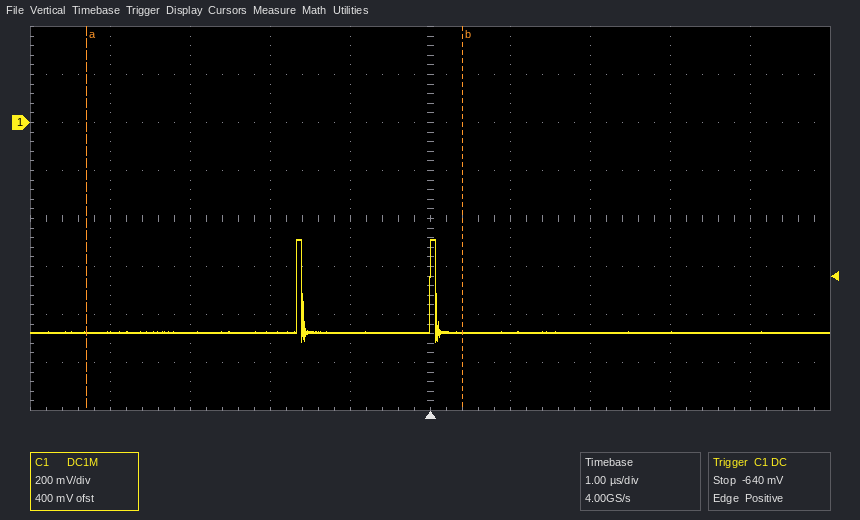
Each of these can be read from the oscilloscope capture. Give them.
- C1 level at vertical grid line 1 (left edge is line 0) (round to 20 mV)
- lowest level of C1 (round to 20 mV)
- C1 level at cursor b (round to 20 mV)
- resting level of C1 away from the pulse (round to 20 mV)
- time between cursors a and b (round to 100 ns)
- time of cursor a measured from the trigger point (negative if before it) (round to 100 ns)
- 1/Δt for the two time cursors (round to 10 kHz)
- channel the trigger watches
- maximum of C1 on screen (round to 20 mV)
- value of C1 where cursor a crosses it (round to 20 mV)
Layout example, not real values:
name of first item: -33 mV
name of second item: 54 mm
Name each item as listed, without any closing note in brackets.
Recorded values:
C1 level at vertical grid line 1 (left edge is line 0): -880 mV
lowest level of C1: -920 mV
C1 level at cursor b: -880 mV
resting level of C1 away from the pulse: -880 mV
time between cursors a and b: 4.7 µs
time of cursor a measured from the trigger point (negative if before it): -4.3 µs
1/Δt for the two time cursors: 210 kHz
channel the trigger watches: C1
maximum of C1 on screen: -480 mV
value of C1 where cursor a crosses it: -880 mV
